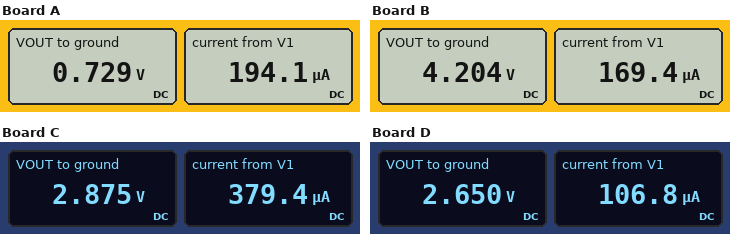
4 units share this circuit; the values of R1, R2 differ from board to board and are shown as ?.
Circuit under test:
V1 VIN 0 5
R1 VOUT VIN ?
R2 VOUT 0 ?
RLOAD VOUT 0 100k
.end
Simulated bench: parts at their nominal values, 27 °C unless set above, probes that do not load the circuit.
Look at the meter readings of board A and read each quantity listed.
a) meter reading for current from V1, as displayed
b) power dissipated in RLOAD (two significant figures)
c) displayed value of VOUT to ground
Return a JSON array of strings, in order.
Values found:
["194.1 µA", "5.3 µW", "0.729 V"]
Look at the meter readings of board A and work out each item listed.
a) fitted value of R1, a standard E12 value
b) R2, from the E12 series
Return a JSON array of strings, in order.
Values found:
["22 kΩ", "3.9 kΩ"]
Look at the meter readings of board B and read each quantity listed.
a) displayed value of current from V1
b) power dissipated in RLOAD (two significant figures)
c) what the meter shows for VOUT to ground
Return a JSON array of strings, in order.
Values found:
["169.4 µA", "180 µW", "4.204 V"]
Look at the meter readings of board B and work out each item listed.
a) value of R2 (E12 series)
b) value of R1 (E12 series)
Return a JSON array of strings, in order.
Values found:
["33 kΩ", "4.7 kΩ"]
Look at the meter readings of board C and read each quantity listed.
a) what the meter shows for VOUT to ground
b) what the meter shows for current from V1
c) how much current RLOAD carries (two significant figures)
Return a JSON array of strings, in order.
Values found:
["2.875 V", "379.4 µA", "29 µA"]
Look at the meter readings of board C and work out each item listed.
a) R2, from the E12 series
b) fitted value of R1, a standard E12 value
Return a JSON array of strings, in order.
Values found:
["8.2 kΩ", "5.6 kΩ"]
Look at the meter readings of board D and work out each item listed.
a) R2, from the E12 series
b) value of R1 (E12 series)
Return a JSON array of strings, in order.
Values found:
["33 kΩ", "22 kΩ"]
